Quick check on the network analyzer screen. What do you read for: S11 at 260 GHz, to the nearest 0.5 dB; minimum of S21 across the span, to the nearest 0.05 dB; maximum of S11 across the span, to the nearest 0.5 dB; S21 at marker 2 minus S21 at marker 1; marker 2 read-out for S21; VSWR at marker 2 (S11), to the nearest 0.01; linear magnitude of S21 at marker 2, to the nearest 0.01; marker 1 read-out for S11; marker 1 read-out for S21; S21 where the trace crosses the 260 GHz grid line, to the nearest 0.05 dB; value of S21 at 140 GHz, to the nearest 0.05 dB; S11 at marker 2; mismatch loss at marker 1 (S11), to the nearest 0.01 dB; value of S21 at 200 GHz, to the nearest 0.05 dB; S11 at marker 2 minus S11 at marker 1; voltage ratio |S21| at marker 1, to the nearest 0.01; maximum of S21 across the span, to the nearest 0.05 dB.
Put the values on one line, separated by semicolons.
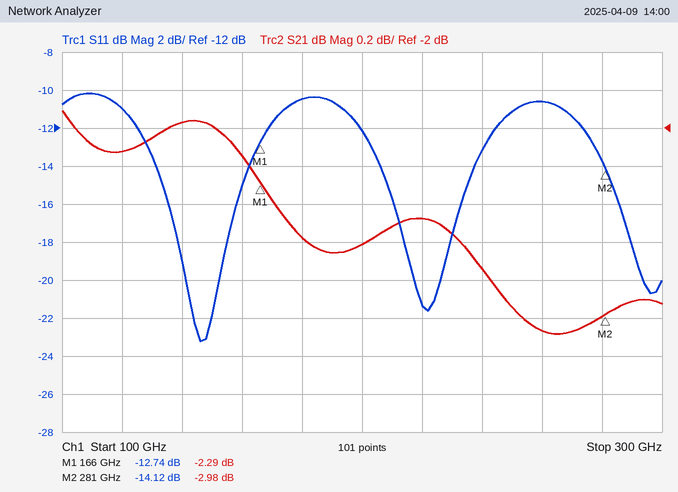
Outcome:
-10.5 dB; -3.10 dB; -10.0 dB; -0.69 dB; -2.98 dB; 1.49; 0.71; -12.74 dB; -2.29 dB; -3.05 dB; -1.95 dB; -14.12 dB; 0.24 dB; -2.60 dB; -1.38 dB; 0.77; -1.90 dB
